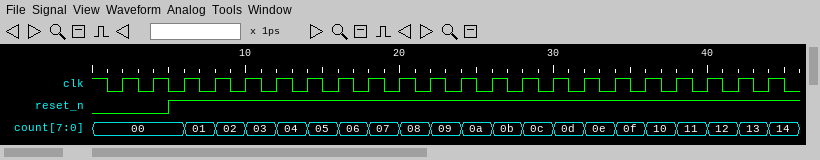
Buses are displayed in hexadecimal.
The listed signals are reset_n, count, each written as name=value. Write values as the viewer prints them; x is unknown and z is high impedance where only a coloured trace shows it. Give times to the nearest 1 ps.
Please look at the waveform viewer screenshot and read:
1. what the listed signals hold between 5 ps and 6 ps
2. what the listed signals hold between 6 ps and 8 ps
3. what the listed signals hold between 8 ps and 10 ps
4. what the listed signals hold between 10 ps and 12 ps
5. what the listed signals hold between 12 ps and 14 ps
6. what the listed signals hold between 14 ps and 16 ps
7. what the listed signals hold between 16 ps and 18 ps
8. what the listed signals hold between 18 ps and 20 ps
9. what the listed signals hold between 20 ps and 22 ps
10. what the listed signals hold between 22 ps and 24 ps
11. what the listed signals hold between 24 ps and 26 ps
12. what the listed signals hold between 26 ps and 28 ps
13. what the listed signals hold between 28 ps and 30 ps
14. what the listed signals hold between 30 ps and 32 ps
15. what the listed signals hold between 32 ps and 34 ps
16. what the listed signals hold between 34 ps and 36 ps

reset_n=1, count=00
reset_n=1, count=01
reset_n=1, count=02
reset_n=1, count=03
reset_n=1, count=04
reset_n=1, count=05
reset_n=1, count=06
reset_n=1, count=07
reset_n=1, count=08
reset_n=1, count=09
reset_n=1, count=0a
reset_n=1, count=0b
reset_n=1, count=0c
reset_n=1, count=0d
reset_n=1, count=0e
reset_n=1, count=0f
